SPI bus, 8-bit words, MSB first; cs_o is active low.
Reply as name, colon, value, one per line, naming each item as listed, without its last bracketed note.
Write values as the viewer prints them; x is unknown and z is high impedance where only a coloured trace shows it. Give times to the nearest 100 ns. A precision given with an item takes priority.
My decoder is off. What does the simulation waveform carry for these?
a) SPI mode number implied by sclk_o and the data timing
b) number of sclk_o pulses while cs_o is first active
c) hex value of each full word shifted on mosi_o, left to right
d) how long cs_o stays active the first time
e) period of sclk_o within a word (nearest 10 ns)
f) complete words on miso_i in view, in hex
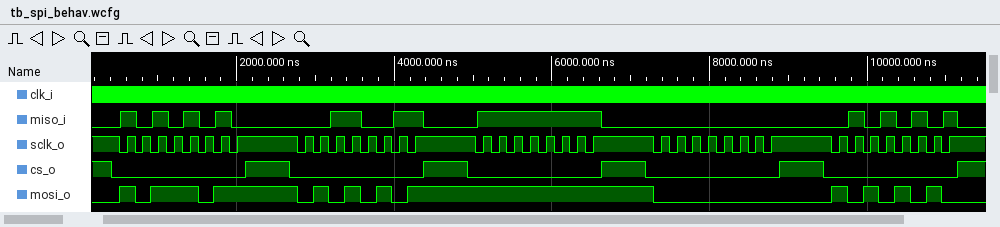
SPI mode number implied by sclk_o and the data timing: 3
number of sclk_o pulses while cs_o is first active: 8
hex value of each full word shifted on mosi_o, left to right: BB, 55, FF, 00, AA
how long cs_o stays active the first time: 1700 ns
period of sclk_o within a word: 200 ns
complete words on miso_i in view, in hex: AA, 33, FF, 00, 55
